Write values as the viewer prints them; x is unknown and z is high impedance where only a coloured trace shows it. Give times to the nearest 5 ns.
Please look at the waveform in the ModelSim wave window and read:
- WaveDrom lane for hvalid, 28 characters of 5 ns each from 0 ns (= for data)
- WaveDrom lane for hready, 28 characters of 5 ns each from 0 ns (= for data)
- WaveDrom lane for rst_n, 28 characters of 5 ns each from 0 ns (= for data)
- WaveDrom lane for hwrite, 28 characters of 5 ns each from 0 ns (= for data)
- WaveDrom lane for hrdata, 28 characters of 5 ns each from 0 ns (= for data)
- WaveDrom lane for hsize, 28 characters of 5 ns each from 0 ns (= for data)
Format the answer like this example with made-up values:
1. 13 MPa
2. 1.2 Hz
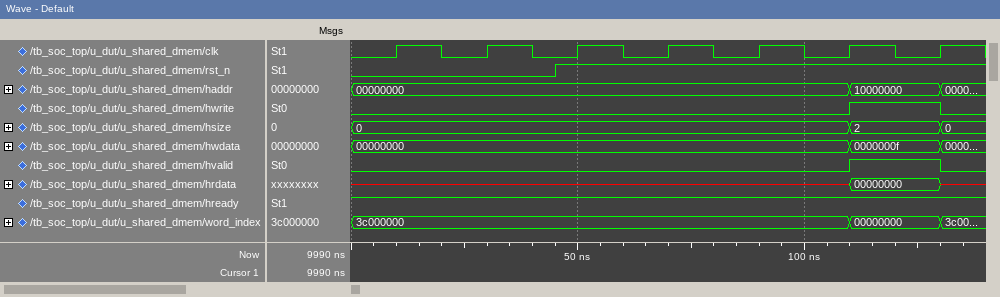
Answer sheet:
1. {name: 'hvalid', wave: '0.....................1...0.'}
2. {name: 'hready', wave: '1...........................'}
3. {name: 'rst_n', wave: '0........1..................'}
4. {name: 'hwrite', wave: '0.....................1...0.'}
5. {name: 'hrdata', wave: 'x.....................=...x.', data: '00000000'}
6. {name: 'hsize', wave: '=.....................=...=.', data: '0 2 0'}
